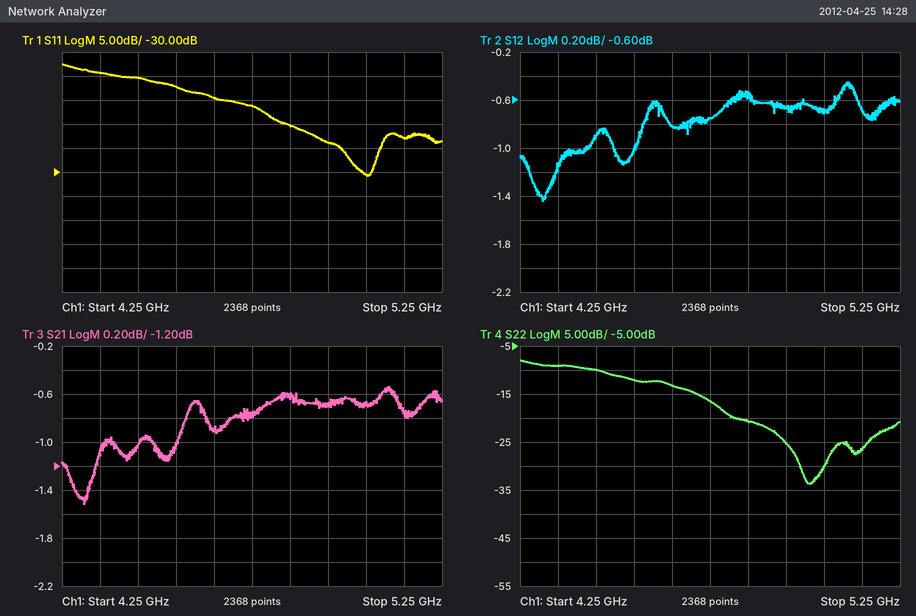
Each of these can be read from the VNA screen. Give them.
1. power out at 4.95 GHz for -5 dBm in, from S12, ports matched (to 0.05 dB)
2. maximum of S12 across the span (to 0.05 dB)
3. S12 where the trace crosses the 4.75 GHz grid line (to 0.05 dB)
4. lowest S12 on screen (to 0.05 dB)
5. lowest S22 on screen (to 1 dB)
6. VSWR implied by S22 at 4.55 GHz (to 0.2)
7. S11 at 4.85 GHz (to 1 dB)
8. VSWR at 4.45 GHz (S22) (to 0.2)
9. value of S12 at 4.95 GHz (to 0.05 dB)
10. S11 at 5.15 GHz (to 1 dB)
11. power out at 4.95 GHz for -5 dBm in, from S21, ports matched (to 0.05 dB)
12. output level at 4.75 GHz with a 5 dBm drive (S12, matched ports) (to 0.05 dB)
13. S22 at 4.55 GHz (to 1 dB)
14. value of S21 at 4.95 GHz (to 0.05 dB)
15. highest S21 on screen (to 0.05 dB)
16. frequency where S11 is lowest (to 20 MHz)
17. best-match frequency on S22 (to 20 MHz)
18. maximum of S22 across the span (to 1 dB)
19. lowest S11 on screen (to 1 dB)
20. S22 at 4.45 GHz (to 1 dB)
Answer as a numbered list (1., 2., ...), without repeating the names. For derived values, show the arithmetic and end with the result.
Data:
1. -5 dBm + (-0.65 dB) = -5.65 dBm
2. -0.45 dB
3. -0.75 dB
4. -1.45 dB
5. -34 dB
6. |Γ| = 10^(-12/20) = 0.2512; VSWR = (1 + 0.2512)/(1 − 0.2512) ≈ 1.67, so 1.6 to the nearest 0.2
7. -20 dB
8. |Γ| = 10^(-10/20) = 0.3162; VSWR = (1 + 0.3162)/(1 − 0.3162) ≈ 1.92, so 2.0 to the nearest 0.2
9. -0.65 dB
10. -23 dB
11. -5 dBm + (-0.70 dB) = -5.70 dBm
12. 5 dBm + (-0.75 dB) = 4.25 dBm
13. -12 dB
14. -0.70 dB
15. -0.55 dB
16. 5.06 GHz
17. 5.02 GHz
18. -8 dB
19. -31 dB
20. -10 dB
